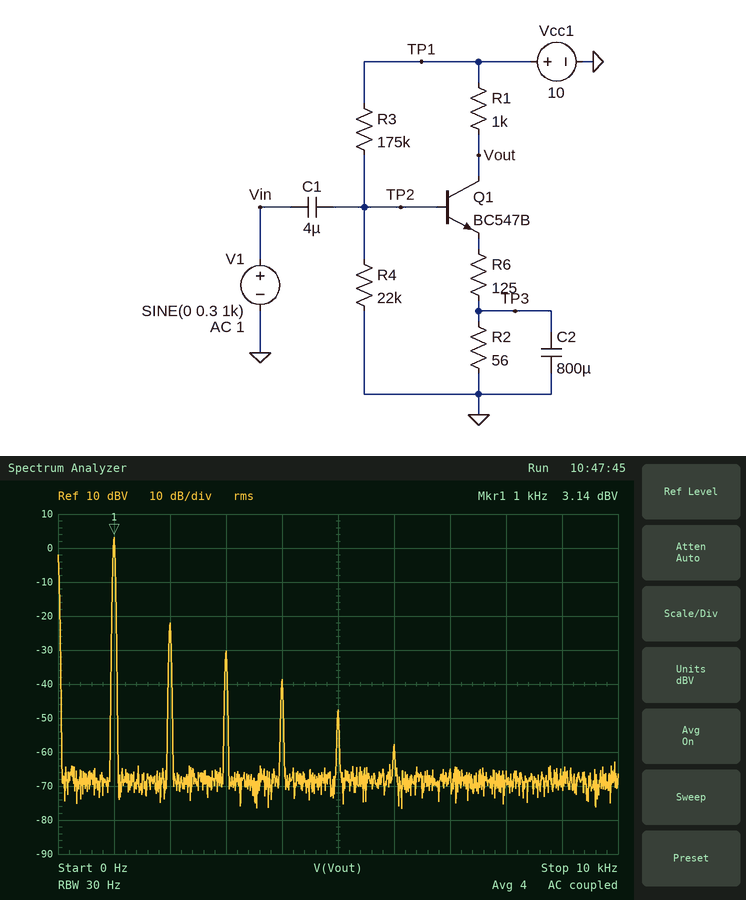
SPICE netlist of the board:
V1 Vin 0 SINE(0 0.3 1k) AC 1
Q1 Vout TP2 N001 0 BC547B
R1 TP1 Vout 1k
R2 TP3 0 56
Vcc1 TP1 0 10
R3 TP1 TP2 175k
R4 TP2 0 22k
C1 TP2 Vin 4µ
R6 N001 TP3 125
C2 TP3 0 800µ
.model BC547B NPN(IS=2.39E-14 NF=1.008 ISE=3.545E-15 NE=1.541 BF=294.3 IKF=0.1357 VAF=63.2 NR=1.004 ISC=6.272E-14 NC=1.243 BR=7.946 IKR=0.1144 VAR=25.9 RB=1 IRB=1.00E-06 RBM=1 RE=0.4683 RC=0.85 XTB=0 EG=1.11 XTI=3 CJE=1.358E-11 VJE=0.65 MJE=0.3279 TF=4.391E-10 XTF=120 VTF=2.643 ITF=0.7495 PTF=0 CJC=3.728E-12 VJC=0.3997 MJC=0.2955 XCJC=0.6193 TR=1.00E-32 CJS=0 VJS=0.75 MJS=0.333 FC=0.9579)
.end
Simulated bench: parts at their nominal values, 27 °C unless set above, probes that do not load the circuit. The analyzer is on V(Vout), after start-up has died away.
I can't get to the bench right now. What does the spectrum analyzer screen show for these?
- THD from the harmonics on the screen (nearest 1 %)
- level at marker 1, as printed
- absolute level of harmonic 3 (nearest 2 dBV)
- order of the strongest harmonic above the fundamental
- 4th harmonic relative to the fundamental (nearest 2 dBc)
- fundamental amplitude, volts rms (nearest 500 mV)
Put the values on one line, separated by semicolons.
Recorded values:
6 %; 3.14 dBV; -30 dBV; 2; -42 dBc; 1.5 V
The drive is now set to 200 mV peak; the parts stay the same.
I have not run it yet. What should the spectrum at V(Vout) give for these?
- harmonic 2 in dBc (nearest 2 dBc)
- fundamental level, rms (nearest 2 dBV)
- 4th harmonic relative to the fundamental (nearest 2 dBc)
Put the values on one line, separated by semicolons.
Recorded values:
-32 dBc; 0 dBV; -58 dBc
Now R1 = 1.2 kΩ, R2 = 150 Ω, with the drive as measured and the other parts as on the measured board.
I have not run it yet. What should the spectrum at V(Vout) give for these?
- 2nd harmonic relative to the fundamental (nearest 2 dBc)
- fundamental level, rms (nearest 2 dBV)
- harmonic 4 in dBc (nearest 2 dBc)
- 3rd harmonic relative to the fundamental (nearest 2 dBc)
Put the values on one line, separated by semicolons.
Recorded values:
-18 dBc; 4 dBV; -38 dBc; -26 dBc
